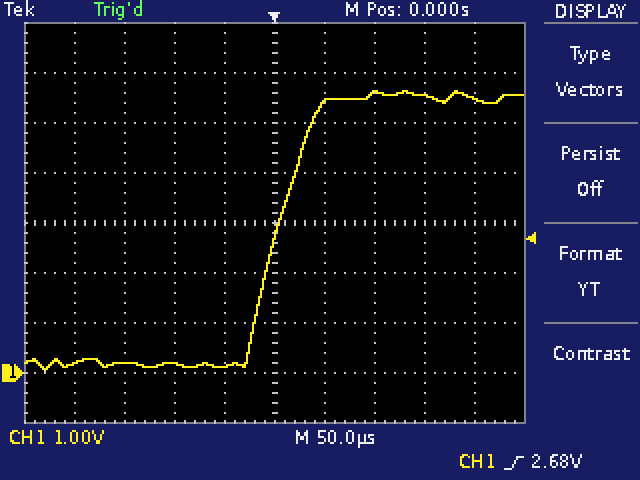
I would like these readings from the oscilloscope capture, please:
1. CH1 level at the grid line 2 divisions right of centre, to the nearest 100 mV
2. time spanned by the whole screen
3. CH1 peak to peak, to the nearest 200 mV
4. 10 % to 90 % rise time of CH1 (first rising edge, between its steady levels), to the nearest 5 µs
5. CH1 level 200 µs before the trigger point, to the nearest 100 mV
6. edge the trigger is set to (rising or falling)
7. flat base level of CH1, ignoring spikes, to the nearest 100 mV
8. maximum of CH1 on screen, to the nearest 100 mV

5.6 V
500 µs
5.6 V
60 µs
200 mV
rising
200 mV
5.6 V
